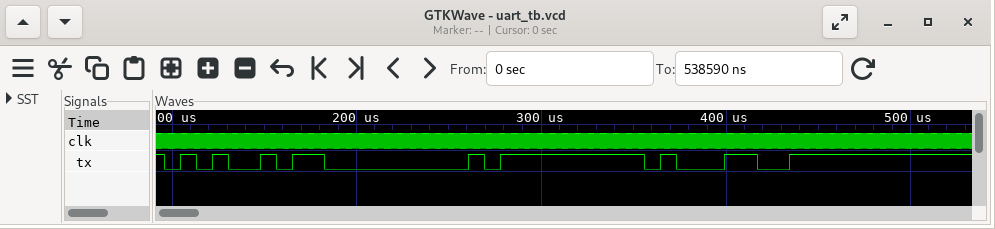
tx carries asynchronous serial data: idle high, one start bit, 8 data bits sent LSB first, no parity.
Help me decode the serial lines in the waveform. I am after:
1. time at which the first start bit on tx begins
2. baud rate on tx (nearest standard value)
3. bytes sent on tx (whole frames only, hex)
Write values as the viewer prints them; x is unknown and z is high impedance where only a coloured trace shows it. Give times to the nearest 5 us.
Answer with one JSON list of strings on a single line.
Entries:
["95 us", "115200 baud", "A5, 00, FF, 31"]
